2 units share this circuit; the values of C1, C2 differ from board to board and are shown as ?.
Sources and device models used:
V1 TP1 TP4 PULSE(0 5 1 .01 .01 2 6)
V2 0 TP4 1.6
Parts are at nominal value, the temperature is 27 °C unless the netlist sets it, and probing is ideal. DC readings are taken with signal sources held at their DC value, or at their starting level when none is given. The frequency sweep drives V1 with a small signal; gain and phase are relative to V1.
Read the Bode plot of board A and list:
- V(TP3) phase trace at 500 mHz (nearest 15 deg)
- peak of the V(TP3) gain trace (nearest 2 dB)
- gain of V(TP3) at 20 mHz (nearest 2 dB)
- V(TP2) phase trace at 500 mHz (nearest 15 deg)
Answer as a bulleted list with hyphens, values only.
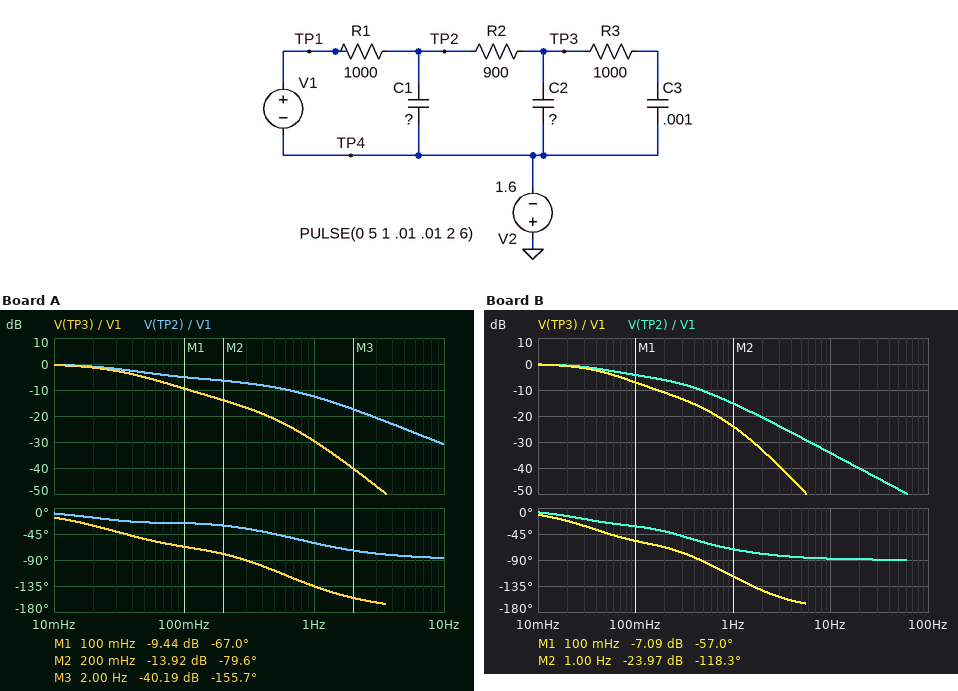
- -105 deg
- 0 dB
- -2 dB
- -45 deg
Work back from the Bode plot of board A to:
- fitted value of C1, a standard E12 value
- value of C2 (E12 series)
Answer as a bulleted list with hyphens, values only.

- 560 µF
- 1.2 mF
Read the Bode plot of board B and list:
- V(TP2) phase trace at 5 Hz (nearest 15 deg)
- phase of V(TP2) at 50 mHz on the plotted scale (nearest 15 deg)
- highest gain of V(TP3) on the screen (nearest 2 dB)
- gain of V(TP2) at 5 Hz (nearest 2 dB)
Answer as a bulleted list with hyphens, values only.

- -90 deg
- -30 deg
- 0 dB
- -28 dB
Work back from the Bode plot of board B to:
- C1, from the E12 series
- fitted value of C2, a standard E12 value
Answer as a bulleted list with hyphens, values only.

- 820 µF
- 330 µF
